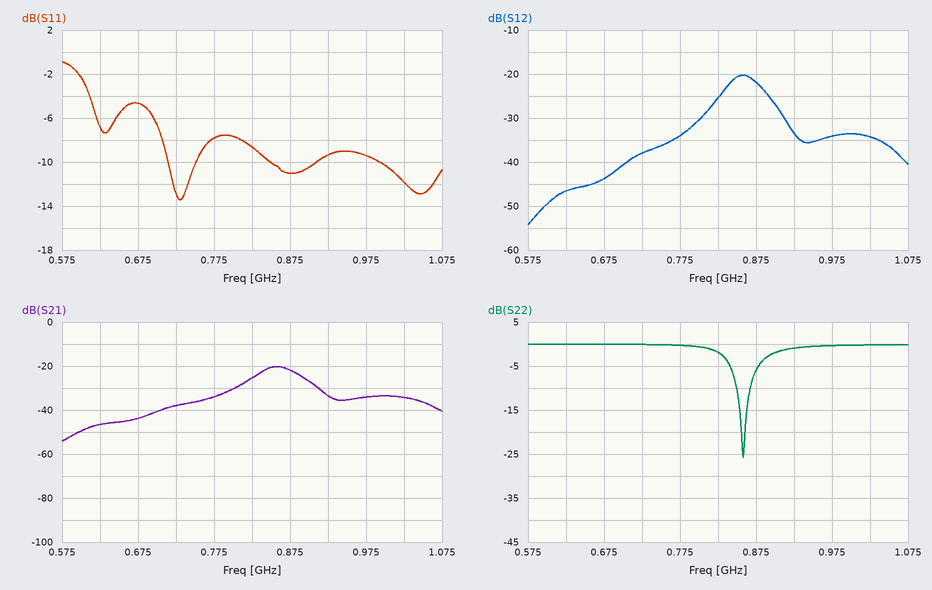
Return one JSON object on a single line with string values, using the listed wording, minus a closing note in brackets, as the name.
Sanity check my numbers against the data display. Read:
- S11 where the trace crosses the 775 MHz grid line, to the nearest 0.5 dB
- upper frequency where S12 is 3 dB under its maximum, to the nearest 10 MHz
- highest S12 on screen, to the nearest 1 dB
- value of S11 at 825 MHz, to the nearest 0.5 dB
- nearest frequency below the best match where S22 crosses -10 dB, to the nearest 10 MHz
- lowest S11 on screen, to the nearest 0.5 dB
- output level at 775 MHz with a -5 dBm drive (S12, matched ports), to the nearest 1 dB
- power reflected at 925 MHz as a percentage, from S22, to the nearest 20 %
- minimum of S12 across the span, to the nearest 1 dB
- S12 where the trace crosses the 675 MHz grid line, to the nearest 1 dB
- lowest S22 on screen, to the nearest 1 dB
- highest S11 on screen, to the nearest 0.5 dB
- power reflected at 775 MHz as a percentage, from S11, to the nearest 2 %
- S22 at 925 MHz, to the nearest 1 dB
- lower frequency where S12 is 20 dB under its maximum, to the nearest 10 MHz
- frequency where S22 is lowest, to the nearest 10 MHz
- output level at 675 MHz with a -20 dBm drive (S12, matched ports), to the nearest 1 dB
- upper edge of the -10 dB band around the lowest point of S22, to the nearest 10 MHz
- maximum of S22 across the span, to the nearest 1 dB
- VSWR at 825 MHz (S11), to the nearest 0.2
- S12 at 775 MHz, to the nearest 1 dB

{"S11 where the trace crosses the 775 MHz grid line, to the nearest 0.5 dB": "-8.0 dB", "upper frequency where S12 is 3 dB under its maximum, to the nearest 10 MHz": "880 MHz", "highest S12 on screen, to the nearest 1 dB": "-20 dB", "value of S11 at 825 MHz, to the nearest 0.5 dB": "-8.5 dB", "nearest frequency below the best match where S22 crosses -10 dB, to the nearest 10 MHz": "850 MHz", "lowest S11 on screen, to the nearest 0.5 dB": "-13.5 dB", "output level at 775 MHz with a -5 dBm drive (S12, matched ports), to the nearest 1 dB": "-39 dBm", "power reflected at 925 MHz as a percentage, from S22, to the nearest 20 %": "80 %", "minimum of S12 across the span, to the nearest 1 dB": "-54 dB", "S12 where the trace crosses the 675 MHz grid line, to the nearest 1 dB": "-44 dB", "lowest S22 on screen, to the nearest 1 dB": "-26 dB", "highest S11 on screen, to the nearest 0.5 dB": "-1.0 dB", "power reflected at 775 MHz as a percentage, from S11, to the nearest 2 %": "16 %", "S22 at 925 MHz, to the nearest 1 dB": "-1 dB", "lower frequency where S12 is 20 dB under its maximum, to the nearest 10 MHz": "700 MHz", "frequency where S22 is lowest, to the nearest 10 MHz": "860 MHz", "output level at 675 MHz with a -20 dBm drive (S12, matched ports), to the nearest 1 dB": "-64 dBm", "upper edge of the -10 dB band around the lowest point of S22, to the nearest 10 MHz": "870 MHz", "maximum of S22 across the span, to the nearest 1 dB": "0 dB", "VSWR at 825 MHz (S11), to the nearest 0.2": "2.2", "S12 at 775 MHz, to the nearest 1 dB": "-34 dB"}
